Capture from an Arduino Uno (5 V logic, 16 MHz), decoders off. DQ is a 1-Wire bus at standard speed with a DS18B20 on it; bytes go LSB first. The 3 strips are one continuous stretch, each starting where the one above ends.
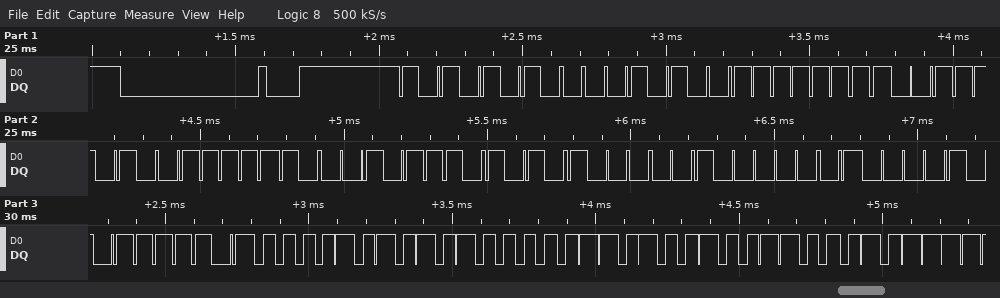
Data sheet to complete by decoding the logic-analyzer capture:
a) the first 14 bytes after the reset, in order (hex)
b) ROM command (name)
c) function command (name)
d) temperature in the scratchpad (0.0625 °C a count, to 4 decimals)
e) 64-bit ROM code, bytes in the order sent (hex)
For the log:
55 28 FF 5C 7E 74 15 04 42 BE 50 05 4B 46
Match ROM
Read Scratchpad
85.0000 °C
28 FF 5C 7E 74 15 04 42
